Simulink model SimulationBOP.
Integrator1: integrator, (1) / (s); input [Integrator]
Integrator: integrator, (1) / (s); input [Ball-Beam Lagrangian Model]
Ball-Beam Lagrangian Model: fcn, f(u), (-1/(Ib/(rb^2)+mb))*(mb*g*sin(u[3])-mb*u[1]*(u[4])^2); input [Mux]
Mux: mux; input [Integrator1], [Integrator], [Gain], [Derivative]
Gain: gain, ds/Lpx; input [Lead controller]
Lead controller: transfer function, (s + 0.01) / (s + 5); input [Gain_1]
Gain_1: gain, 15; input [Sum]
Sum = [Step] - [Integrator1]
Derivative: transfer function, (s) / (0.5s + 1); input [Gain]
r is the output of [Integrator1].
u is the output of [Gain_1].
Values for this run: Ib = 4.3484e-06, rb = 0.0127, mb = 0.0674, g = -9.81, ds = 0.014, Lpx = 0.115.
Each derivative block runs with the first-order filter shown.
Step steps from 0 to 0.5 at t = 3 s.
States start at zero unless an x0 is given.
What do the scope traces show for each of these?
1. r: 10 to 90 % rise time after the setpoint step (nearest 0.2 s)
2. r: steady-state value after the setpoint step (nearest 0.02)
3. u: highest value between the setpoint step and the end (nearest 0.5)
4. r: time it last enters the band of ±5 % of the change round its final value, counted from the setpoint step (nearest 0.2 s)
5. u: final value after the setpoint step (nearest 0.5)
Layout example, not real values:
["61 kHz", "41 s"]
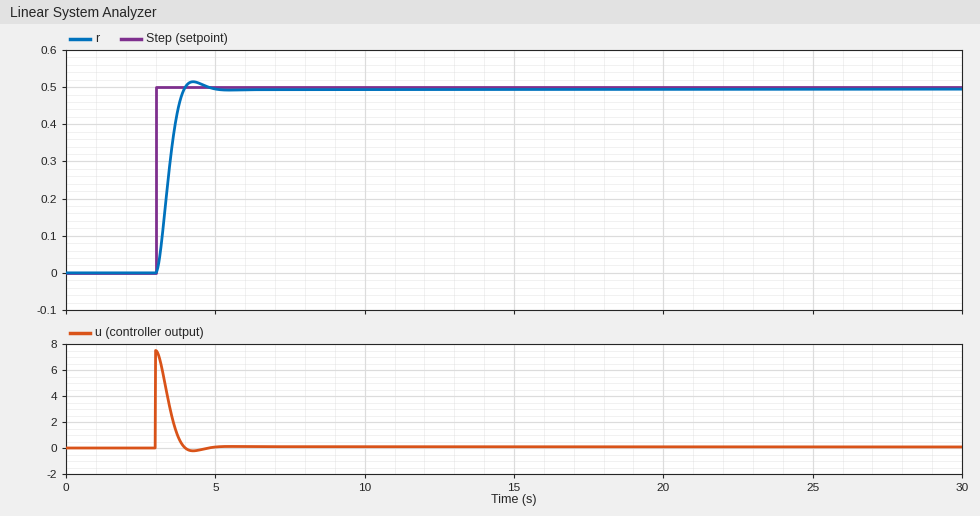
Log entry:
["0.6 s", "0.50", "7.5", "0.8 s", "0.0"]
